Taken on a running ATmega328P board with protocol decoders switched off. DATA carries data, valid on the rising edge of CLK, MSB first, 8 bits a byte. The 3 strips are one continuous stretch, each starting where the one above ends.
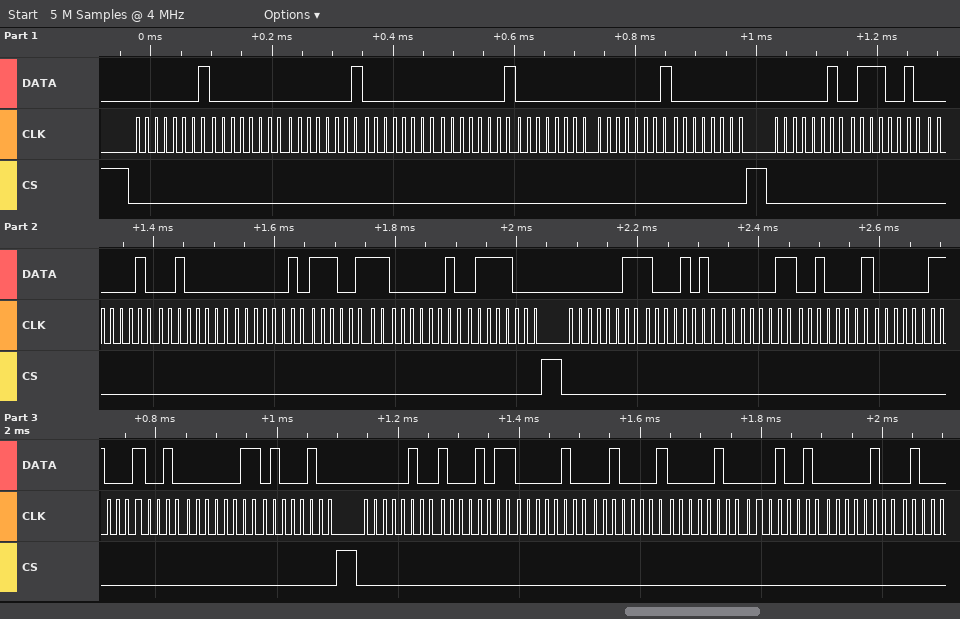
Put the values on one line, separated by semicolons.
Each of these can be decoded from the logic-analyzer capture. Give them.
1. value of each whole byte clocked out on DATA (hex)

01 00 01 00 01 00 01 00 02 72 02 20 02 E7 02 78 03 8A 03 21 03 12 03 44 04 8B 04 21 04 12 04
